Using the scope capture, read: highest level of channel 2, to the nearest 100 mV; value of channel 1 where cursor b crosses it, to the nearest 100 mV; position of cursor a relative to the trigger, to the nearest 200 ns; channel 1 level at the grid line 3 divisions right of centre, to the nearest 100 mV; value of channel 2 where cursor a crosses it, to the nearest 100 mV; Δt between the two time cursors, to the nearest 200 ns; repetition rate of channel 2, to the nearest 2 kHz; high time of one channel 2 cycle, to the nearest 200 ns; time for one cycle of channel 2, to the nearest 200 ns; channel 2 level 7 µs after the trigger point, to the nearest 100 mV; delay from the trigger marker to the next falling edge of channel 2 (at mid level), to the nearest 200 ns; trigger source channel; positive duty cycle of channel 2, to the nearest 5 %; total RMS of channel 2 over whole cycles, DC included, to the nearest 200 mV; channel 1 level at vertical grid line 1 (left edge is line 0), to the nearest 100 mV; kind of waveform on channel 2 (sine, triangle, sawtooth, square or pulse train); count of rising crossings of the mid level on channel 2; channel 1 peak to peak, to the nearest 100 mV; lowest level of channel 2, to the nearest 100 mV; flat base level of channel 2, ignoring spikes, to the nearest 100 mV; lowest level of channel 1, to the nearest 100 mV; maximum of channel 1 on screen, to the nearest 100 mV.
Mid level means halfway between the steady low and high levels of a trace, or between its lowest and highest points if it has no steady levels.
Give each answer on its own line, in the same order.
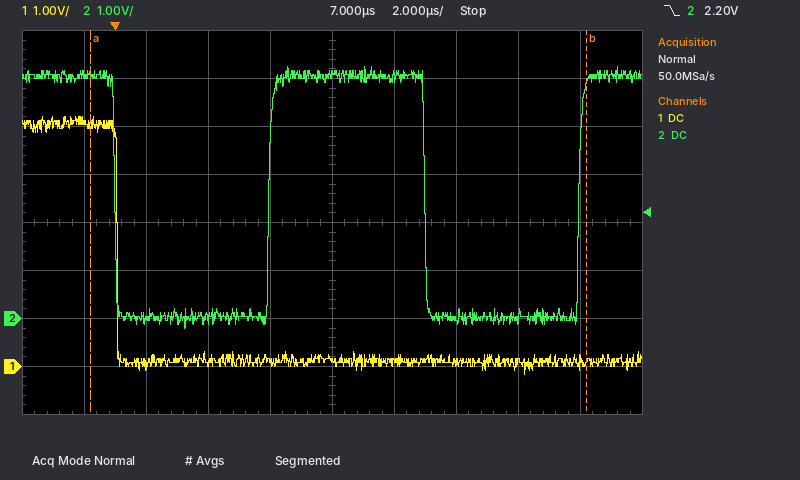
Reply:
5.2 V
100 mV
-800 ns
100 mV
5.1 V
16.0 µs
100 kHz
5.0 µs
10.0 µs
5.1 V
10.0 µs
channel 2
50 %
3.6 V
5.1 V
square
2
5.4 V
-200 mV
0.0 V
-200 mV
5.2 V
